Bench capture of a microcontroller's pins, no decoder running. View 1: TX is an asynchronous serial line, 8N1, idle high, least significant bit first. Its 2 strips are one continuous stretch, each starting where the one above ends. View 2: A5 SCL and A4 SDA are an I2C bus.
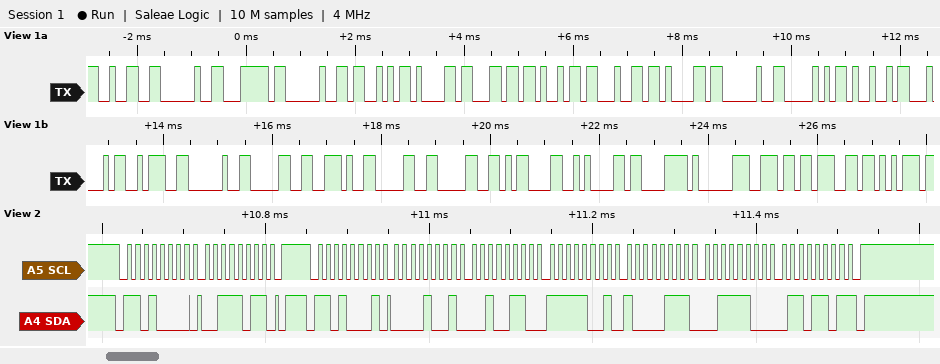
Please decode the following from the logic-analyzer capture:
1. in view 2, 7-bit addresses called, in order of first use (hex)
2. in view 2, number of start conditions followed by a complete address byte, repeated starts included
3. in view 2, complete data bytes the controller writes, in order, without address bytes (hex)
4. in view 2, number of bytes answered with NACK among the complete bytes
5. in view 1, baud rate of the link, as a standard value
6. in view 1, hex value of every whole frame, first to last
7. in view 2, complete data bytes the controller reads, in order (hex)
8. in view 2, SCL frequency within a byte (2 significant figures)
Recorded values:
0x68
2
3B
1
9600 baud
32 20 7C 20 53 61 6C 69 64 61 20 50 49 44 3A 20 30 2E 30 30 0D 0A C3 81 6E 67 75
09 26 F9 87 3C 6D
100 kHz
